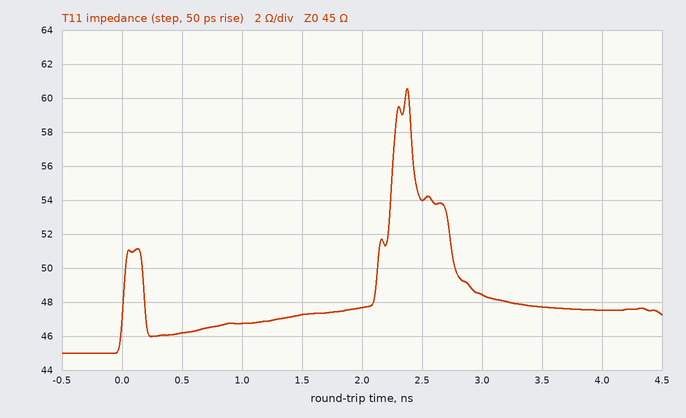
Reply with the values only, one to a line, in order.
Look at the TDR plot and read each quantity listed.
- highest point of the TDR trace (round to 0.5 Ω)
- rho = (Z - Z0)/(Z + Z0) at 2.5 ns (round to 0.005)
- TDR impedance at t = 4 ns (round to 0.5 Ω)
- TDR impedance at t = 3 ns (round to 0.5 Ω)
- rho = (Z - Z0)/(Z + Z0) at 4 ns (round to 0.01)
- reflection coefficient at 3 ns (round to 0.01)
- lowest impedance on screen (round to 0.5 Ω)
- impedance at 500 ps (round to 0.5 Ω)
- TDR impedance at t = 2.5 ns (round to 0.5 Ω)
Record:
60.5 Ω
+0.090
47.5 Ω
48.5 Ω
+0.03
+0.04
45.0 Ω
46.0 Ω
54.0 Ω
